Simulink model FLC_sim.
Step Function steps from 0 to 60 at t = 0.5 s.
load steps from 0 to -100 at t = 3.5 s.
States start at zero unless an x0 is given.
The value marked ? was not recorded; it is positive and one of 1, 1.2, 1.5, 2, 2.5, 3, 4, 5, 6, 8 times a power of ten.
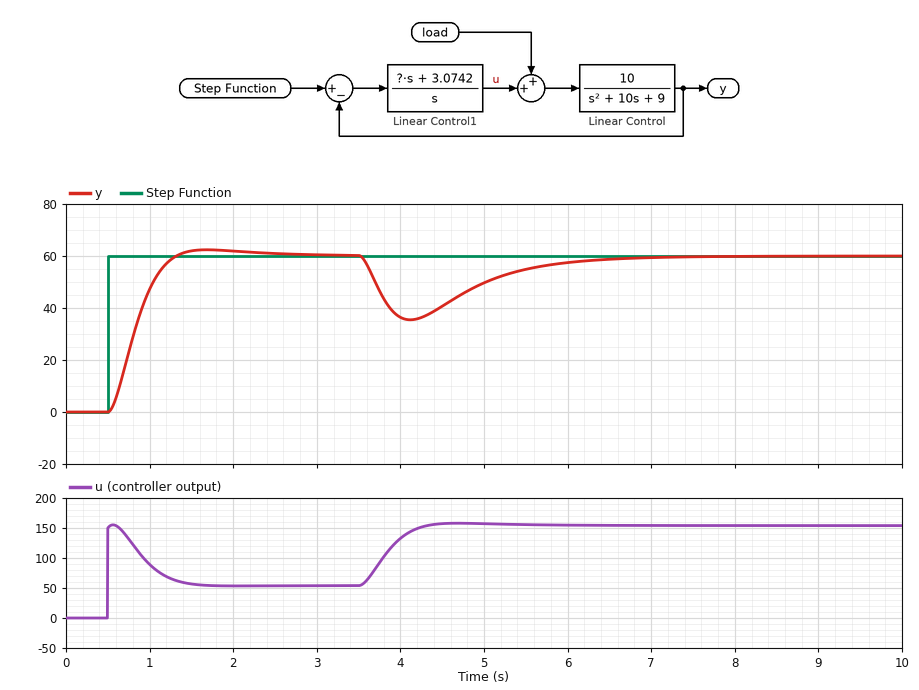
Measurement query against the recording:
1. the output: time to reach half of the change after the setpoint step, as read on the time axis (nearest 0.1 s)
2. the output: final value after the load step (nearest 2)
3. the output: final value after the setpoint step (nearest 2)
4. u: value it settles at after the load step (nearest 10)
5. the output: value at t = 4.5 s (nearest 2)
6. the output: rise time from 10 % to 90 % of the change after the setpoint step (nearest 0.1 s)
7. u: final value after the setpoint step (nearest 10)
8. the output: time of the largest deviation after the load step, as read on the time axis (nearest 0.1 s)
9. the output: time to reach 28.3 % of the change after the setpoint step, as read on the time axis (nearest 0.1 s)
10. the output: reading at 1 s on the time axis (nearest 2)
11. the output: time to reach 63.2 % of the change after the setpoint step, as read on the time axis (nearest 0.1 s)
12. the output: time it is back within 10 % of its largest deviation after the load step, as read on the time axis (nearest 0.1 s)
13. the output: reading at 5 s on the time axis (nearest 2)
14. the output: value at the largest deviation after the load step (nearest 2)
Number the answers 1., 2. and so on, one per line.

1. 0.8 s
2. 60
3. 60
4. 150
5. 40
6. 0.5 s
7. 50
8. 4.1 s
9. 0.7 s
10. 48
11. 0.9 s
12. 6.0 s
13. 50
14. 36
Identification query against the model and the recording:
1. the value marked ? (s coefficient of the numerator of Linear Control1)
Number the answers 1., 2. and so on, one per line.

1. 2.5
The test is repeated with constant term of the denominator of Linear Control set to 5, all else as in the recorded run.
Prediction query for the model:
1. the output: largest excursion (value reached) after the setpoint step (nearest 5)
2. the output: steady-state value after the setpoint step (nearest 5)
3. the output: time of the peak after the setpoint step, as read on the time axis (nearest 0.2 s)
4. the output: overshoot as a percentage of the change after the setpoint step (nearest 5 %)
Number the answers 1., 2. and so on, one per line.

1. 70
2. 60
3. 1.6 s
4. 15 %
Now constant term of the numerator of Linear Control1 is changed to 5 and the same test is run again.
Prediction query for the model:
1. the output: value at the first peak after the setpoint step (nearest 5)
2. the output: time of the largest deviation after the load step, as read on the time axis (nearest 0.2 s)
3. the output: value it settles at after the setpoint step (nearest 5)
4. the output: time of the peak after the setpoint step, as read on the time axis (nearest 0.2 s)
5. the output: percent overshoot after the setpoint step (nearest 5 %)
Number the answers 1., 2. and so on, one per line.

1. 70
2. 4.0 s
3. 60
4. 1.4 s
5. 15 %
